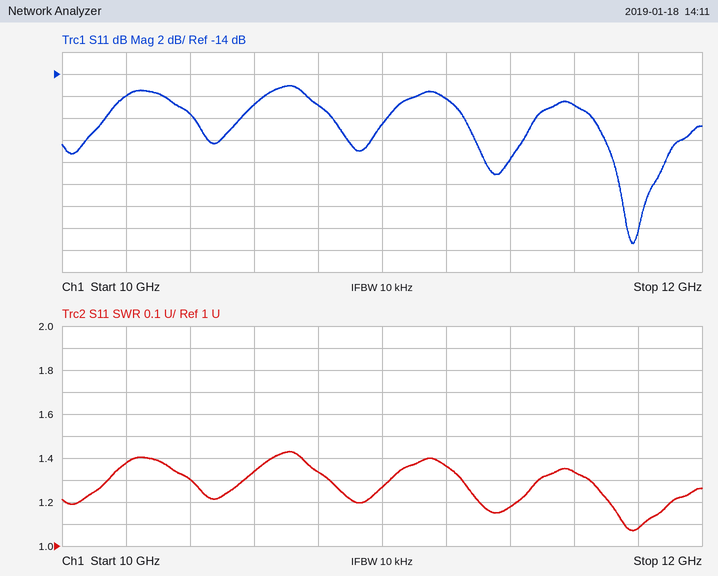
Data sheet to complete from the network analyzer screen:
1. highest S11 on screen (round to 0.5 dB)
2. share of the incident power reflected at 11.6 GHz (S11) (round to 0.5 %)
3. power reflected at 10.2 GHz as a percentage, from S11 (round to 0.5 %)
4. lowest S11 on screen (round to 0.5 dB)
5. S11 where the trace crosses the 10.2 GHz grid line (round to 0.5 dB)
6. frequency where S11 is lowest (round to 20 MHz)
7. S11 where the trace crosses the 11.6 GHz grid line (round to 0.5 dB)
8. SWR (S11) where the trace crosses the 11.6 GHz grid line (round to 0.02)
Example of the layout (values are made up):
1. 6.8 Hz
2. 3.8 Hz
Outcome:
1. -15.0 dB
2. 2.0 %
3. 2.5 %
4. -29.5 dB
5. -16.0 dB
6. 11.78 GHz
7. -17.0 dB
8. 1.34
